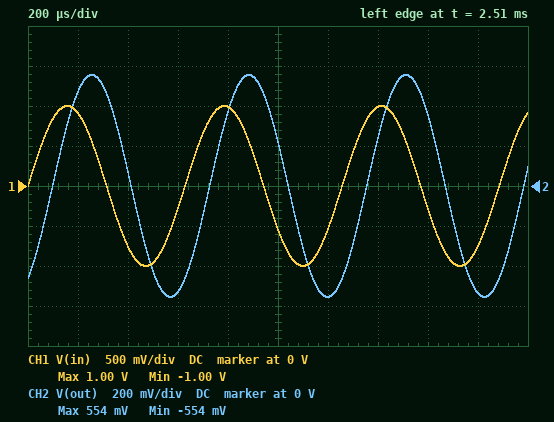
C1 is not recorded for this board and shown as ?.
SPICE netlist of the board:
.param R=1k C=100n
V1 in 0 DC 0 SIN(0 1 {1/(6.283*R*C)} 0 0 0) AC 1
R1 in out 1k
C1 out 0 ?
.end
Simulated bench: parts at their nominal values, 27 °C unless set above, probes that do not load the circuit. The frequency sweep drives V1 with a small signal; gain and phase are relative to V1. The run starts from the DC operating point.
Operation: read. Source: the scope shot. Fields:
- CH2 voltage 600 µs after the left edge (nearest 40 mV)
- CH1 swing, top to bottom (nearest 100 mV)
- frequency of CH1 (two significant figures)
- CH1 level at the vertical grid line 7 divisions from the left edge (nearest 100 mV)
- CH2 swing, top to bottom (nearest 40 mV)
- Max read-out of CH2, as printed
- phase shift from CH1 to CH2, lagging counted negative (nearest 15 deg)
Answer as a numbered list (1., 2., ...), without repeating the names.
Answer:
1. -520 mV
2. 2.0 V
3. 1.6 kHz
4. 1.0 V
5. 1.12 V
6. 554 mV
7. -60 deg
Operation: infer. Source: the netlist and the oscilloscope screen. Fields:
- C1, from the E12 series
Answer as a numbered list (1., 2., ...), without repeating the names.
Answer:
1. 150 nF
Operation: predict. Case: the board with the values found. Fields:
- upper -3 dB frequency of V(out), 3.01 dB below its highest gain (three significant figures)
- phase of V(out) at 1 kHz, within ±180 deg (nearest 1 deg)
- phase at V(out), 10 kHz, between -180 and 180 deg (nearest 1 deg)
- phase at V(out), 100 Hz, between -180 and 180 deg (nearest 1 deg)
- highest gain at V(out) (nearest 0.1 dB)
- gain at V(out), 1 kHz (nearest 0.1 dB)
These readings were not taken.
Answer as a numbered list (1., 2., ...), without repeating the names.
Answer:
1. 1.06 kHz
2. -43 deg
3. -84 deg
4. -5 deg
5. 0 dB
6. -2.8 dB
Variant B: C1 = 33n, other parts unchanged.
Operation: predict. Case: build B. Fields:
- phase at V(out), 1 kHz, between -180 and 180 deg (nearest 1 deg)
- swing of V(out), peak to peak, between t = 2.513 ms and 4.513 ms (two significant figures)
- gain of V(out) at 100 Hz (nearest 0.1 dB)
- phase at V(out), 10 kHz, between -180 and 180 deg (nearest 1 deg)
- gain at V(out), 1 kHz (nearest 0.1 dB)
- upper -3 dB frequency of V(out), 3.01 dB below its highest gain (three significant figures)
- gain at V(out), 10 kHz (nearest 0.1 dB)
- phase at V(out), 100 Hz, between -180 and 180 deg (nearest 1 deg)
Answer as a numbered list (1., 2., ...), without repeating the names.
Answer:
1. -12 deg
2. 1.9 V
3. 0 dB
4. -64 deg
5. -0.2 dB
6. 4.82 kHz
7. -7.2 dB
8. -1 deg
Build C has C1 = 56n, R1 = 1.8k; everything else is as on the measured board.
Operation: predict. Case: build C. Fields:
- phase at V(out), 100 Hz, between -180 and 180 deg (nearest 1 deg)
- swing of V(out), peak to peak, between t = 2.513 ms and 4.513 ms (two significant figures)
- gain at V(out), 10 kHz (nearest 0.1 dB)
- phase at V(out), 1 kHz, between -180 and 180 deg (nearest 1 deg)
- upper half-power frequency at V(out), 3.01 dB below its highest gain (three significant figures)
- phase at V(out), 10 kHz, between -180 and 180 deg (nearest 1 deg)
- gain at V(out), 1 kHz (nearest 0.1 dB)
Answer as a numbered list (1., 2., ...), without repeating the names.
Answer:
1. -4 deg
2. 1.4 V
3. -16.1 dB
4. -32 deg
5. 1.58 kHz
6. -81 deg
7. -1.5 dB
